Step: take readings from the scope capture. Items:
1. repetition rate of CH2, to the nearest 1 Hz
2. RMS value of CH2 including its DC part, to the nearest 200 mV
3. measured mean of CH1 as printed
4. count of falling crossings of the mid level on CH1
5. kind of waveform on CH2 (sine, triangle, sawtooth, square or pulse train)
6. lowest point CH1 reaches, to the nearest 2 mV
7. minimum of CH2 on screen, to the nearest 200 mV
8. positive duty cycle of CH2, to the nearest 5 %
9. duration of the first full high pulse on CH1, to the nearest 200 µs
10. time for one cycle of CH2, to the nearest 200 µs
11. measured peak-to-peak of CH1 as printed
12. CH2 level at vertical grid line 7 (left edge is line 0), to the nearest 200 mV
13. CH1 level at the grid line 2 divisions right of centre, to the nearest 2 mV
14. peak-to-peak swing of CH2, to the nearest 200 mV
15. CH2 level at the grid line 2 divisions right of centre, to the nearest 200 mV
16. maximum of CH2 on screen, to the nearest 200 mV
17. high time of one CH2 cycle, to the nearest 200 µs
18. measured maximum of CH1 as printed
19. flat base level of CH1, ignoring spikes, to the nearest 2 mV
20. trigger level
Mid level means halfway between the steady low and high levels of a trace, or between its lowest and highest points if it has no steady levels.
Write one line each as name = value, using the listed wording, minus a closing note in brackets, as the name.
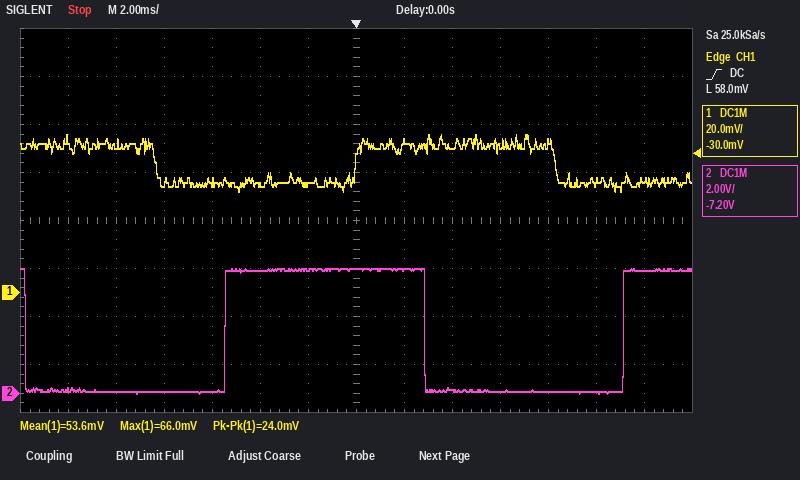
repetition rate of CH2, to the nearest 1 Hz = 60 Hz
RMS value of CH2 including its DC part, to the nearest 200 mV = 3.6 V
measured mean of CH1 as printed = 53.6 mV
count of falling crossings of the mid level on CH1 = 2
kind of waveform on CH2 = square
lowest point CH1 reaches, to the nearest 2 mV = 42 mV
minimum of CH2 on screen, to the nearest 200 mV = 0.0 V
positive duty cycle of CH2, to the nearest 5 % = 50 %
duration of the first full high pulse on CH1, to the nearest 200 µs = 8.4 ms
time for one cycle of CH2, to the nearest 200 µs = 16.6 ms
measured peak-to-peak of CH1 as printed = 24.0 mV
CH2 level at vertical grid line 7 (left edge is line 0), to the nearest 200 mV = 5.2 V
CH1 level at the grid line 2 divisions right of centre, to the nearest 2 mV = 60 mV
peak-to-peak swing of CH2, to the nearest 200 mV = 5.2 V
CH2 level at the grid line 2 divisions right of centre, to the nearest 200 mV = 200 mV
maximum of CH2 on screen, to the nearest 200 mV = 5.2 V
high time of one CH2 cycle, to the nearest 200 µs = 8.4 ms
measured maximum of CH1 as printed = 66.0 mV
flat base level of CH1, ignoring spikes, to the nearest 2 mV = 46 mV
trigger level = 58.0 mV
